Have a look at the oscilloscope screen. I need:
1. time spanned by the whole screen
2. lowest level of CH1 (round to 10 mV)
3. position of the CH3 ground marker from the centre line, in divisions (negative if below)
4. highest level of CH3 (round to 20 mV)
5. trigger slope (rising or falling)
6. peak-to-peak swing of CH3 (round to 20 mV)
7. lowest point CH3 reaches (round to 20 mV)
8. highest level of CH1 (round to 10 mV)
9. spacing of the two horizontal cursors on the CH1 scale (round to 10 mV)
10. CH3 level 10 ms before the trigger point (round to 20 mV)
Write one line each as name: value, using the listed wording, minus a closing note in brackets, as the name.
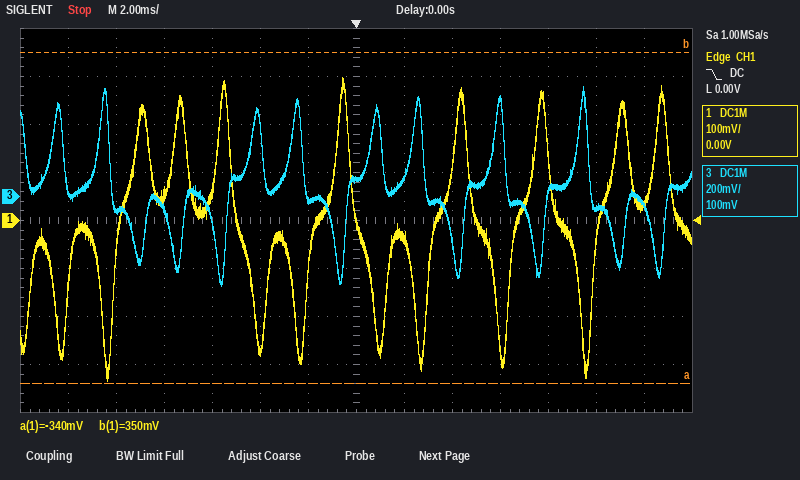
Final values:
time spanned by the whole screen: 28 ms
lowest level of CH1: -340 mV
position of the CH3 ground marker from the centre line, in divisions: +0.5 div
highest level of CH3: 460 mV
trigger slope: falling
peak-to-peak swing of CH3: 840 mV
lowest point CH3 reaches: -380 mV
highest level of CH1: 300 mV
spacing of the two horizontal cursors on the CH1 scale: 690 mV
CH3 level 10 ms before the trigger point: -60 mV
